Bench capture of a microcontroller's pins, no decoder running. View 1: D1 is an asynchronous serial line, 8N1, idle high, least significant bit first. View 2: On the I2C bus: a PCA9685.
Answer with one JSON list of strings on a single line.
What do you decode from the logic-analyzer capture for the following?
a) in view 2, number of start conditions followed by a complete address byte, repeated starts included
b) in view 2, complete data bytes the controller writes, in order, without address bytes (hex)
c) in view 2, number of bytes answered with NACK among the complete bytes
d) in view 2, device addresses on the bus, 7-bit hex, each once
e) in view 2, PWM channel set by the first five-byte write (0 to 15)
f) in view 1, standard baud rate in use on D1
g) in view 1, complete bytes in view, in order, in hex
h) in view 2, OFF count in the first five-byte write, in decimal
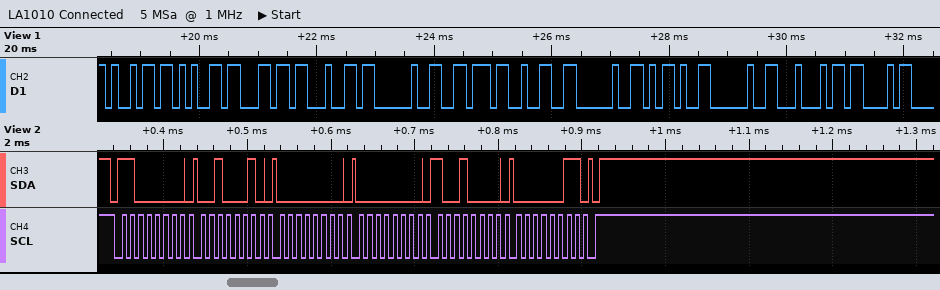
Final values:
["1", "22 00 00 90 03", "0", "0x60", "7", "9600 baud", "69 65 6C 64 20 76 32 20 2D 20 44 43", "912"]
